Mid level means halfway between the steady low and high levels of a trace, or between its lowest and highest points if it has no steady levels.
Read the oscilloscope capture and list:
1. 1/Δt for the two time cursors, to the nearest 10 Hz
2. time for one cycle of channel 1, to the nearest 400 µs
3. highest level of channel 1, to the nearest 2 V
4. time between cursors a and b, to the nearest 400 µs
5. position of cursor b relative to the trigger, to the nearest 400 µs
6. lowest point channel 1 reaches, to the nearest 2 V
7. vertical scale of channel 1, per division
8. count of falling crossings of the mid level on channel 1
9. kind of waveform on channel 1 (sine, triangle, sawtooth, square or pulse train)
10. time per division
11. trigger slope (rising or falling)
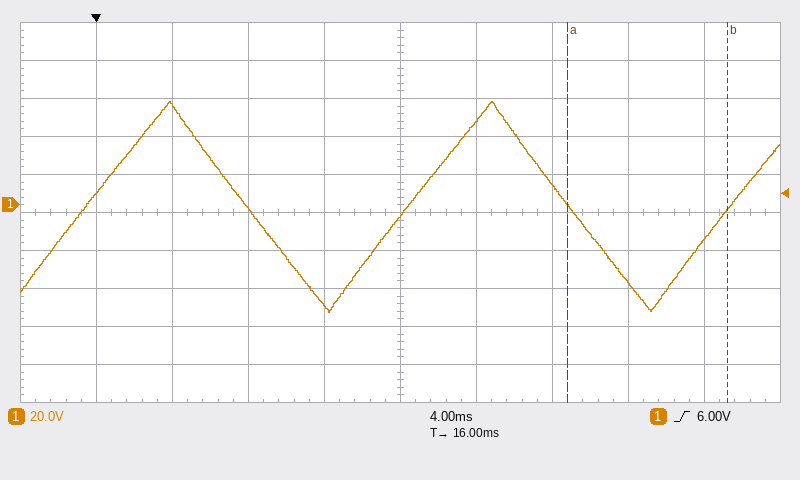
120 Hz
16.8 ms
54 V
8.4 ms
+33.2 ms
-56 V
20 V
2
triangle
4 ms
rising
